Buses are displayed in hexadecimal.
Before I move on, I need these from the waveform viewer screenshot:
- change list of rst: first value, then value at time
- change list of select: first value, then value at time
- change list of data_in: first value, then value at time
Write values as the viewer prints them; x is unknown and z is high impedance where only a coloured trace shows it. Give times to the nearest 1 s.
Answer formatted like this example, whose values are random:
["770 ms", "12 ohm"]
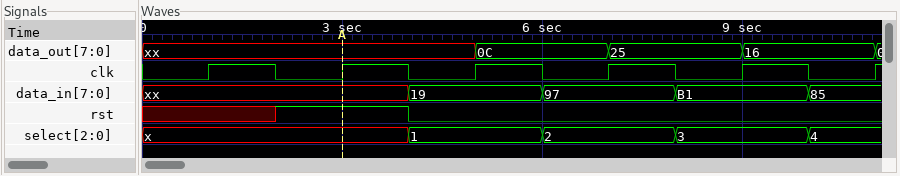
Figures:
["x, 1 at 2 s, 0 at 4 s", "x, 1 at 4 s, 2 at 6 s, 3 at 8 s, 4 at 10 s", "xx, 19 at 4 s, 97 at 6 s, B1 at 8 s, 85 at 10 s"]
